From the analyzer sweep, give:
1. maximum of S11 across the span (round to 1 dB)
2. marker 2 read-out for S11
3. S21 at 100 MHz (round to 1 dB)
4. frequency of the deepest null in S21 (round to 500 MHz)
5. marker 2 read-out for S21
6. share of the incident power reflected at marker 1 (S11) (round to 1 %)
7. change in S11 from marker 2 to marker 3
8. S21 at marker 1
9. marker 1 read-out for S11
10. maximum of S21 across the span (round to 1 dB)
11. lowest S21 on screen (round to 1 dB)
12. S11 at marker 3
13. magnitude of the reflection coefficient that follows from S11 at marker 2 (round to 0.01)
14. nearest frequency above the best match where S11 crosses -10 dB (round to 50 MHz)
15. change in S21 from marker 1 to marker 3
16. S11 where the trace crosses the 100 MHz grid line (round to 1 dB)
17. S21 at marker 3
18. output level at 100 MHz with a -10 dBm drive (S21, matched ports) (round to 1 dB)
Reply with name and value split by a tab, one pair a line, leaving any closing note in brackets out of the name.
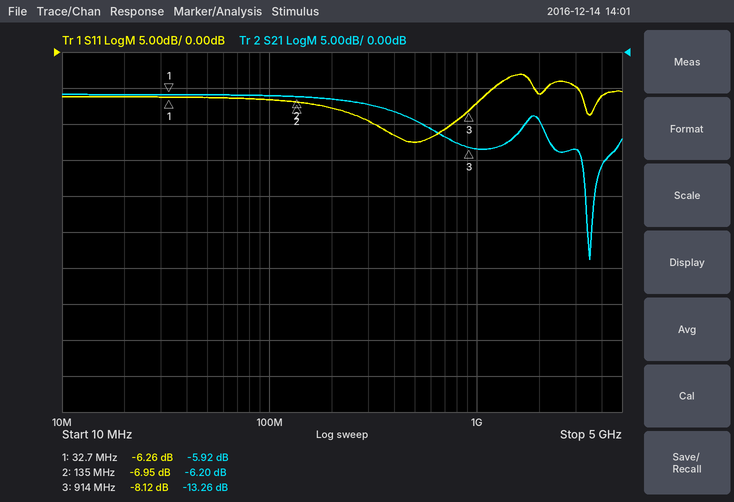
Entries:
maximum of S11 across the span	-3 dB
marker 2 read-out for S11	-6.95 dB
S21 at 100 MHz	-6 dB
frequency of the deepest null in S21	3.5 GHz
marker 2 read-out for S21	-6.20 dB
share of the incident power reflected at marker 1 (S11)	24 %
change in S11 from marker 2 to marker 3	-1.17 dB
S21 at marker 1	-5.92 dB
marker 1 read-out for S11	-6.26 dB
maximum of S21 across the span	-6 dB
lowest S21 on screen	-29 dB
S11 at marker 3	-8.12 dB
magnitude of the reflection coefficient that follows from S11 at marker 2	0.45
nearest frequency above the best match where S11 crosses -10 dB	750 MHz
change in S21 from marker 1 to marker 3	-7.34 dB
S11 where the trace crosses the 100 MHz grid line	-7 dB
S21 at marker 3	-13.26 dB
output level at 100 MHz with a -10 dBm drive (S21, matched ports)	-16 dBm
